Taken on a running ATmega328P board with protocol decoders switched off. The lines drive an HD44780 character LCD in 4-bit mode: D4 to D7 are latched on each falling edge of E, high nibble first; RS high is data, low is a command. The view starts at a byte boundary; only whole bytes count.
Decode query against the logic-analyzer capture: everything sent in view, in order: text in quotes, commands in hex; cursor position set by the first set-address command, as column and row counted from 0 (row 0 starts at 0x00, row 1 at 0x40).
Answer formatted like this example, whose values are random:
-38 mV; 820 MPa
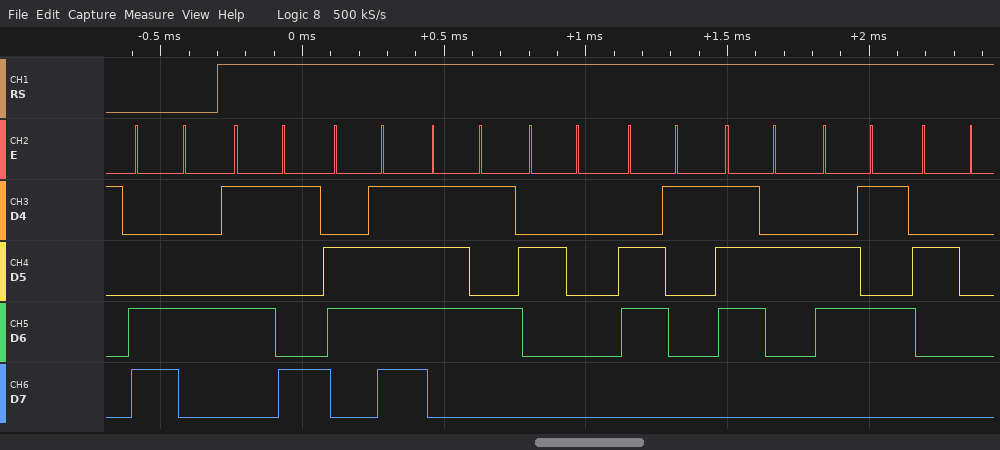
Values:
0xC4 "You are "; column 4, row 1
